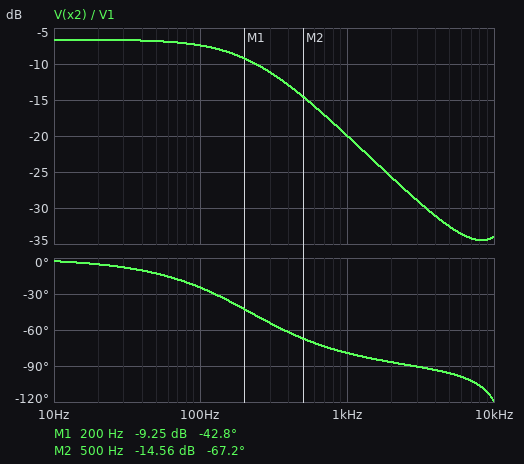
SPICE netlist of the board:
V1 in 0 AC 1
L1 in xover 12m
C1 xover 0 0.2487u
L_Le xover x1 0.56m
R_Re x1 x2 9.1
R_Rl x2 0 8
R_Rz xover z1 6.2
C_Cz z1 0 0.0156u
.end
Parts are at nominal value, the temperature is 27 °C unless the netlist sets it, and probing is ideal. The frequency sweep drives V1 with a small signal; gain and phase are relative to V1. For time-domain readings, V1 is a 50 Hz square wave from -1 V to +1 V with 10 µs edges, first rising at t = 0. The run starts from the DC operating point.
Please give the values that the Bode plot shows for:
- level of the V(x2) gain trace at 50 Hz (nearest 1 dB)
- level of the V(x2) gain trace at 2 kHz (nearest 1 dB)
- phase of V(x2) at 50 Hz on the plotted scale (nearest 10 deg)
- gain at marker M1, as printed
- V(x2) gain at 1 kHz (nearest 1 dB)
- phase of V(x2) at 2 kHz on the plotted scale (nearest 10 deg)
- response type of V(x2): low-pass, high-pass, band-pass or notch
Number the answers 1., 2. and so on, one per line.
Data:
1. -7 dB
2. -26 dB
3. -10 deg
4. -9.25 dB
5. -20 dB
6. -90 deg
7. low-pass
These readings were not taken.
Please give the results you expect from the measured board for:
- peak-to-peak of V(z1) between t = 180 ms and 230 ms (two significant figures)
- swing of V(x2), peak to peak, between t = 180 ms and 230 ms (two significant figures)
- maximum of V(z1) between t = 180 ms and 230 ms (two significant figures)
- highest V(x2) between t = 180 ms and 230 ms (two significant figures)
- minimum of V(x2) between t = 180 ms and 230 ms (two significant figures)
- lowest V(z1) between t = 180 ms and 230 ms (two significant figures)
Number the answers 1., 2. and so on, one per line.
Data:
1. 2.0 V
2. 940 mV
3. 1.0 V
4. 470 mV
5. -470 mV
6. -1.0 V
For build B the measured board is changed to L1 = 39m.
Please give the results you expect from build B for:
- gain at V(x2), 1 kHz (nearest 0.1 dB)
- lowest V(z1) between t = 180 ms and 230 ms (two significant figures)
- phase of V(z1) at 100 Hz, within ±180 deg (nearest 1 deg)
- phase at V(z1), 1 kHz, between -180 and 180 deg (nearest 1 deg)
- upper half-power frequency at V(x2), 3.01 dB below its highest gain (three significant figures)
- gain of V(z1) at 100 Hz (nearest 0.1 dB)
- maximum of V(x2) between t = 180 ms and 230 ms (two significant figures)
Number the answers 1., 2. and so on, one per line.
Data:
1. -29.8 dB
2. -970 mV
3. -54 deg
4. -76 deg
5. 68.9 Hz
6. -4.9 dB
7. 460 mV
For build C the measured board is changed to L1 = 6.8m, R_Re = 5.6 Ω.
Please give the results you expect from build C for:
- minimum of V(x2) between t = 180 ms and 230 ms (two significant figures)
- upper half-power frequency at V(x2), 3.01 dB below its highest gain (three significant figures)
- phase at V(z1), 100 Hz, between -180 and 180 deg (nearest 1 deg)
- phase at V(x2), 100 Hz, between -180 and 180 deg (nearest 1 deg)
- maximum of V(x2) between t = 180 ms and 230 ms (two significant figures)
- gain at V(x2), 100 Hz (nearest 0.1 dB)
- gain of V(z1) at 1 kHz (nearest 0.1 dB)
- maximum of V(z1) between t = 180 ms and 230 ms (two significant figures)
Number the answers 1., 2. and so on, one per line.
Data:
1. -590 mV
2. 296 Hz
3. -17 deg
4. -19 deg
5. 590 mV
6. -5.1 dB
7. -10.6 dB
8. 1.0 V
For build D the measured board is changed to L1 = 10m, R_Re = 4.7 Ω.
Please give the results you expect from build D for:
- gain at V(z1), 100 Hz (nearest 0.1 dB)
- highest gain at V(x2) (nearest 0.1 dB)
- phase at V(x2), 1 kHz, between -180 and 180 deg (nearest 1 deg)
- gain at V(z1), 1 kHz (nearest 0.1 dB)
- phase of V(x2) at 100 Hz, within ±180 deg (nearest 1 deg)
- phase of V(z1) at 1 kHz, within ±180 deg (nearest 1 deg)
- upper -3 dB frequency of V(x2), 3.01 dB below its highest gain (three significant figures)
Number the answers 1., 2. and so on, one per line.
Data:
1. -1.0 dB
2. -4.0 dB
3. -80 deg
4. -14.1 dB
5. -28 deg
6. -65 deg
7. 192 Hz
